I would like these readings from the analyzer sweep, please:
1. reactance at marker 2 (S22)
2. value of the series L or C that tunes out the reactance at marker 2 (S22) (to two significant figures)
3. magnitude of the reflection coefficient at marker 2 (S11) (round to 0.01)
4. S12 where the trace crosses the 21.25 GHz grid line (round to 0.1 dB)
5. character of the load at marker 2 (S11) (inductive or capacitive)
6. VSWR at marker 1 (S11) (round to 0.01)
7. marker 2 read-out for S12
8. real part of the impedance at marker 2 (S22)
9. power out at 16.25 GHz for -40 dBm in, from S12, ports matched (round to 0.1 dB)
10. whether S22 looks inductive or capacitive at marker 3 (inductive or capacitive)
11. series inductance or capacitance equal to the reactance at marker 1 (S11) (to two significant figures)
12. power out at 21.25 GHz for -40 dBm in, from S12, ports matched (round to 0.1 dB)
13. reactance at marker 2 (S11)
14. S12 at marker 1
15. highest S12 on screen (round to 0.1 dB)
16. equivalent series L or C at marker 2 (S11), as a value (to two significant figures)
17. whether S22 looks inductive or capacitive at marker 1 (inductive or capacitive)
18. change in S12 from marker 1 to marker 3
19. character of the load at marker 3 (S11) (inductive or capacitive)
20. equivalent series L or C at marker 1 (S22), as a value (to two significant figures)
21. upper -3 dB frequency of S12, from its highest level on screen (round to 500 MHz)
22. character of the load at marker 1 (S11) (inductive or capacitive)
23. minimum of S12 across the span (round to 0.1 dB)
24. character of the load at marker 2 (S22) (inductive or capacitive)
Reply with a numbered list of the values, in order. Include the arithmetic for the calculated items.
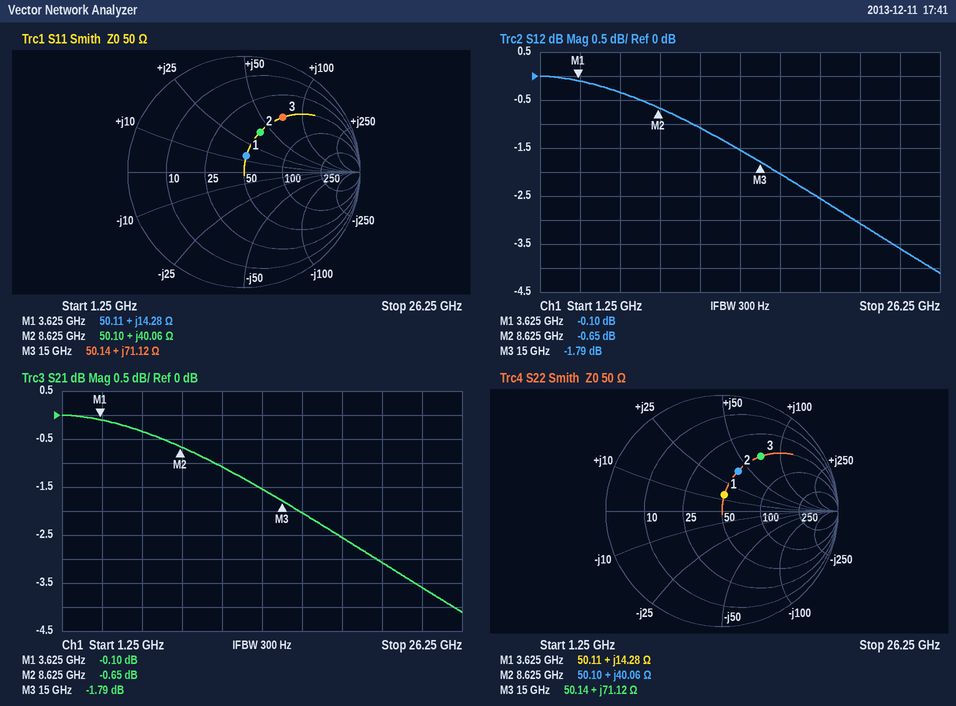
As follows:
1. +40.06 Ω
2. C = 1/(2π × 8.625 GHz × 40.06 Ω) ≈ 461 fF, so 460 fF to two significant figures
3. 0.37
4. -3.1 dB
5. inductive
6. 1.33
7. -0.65 dB
8. 50.10 Ω
9. -40 dBm + (-2.0 dB) = -42.0 dBm
10. inductive
11. L = 14.28 Ω/(2π × 3.625 GHz) ≈ 627 pH, so 630 pH to two significant figures
12. -40 dBm + (-3.1 dB) = -43.1 dBm
13. +40.06 Ω
14. -0.10 dB
15. 0.0 dB
16. L = 40.06 Ω/(2π × 8.625 GHz) ≈ 739 pH, so 740 pH to two significant figures
17. inductive
18. -1.79 − (-0.1) = -1.69 dB
19. inductive
20. L = 14.28 Ω/(2π × 3.625 GHz) ≈ 627 pH, so 630 pH to two significant figures
21. 21.0 GHz
22. inductive
23. -4.1 dB
24. inductive
